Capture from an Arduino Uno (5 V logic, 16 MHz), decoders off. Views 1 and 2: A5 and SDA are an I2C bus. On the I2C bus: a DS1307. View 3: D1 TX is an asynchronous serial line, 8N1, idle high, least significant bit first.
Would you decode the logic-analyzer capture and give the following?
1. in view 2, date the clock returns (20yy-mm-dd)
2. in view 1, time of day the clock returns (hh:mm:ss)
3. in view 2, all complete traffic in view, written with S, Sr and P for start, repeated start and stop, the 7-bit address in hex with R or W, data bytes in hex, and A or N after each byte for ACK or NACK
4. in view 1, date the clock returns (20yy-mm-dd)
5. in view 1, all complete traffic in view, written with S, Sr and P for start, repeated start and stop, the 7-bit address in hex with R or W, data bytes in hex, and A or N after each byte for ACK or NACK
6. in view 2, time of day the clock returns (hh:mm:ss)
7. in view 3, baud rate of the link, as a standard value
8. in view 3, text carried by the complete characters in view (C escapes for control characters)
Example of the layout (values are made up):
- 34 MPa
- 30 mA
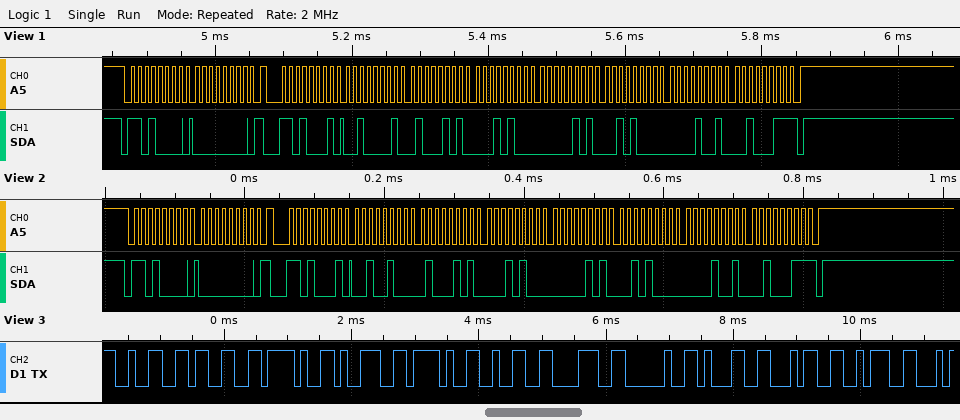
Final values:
- 2023-09-28
- 14:45:21
- S 68W A 00 A Sr 68R A 24 A 45 A 14 A 05 A 28 A 09 A 23 N P
- 2023-09-28
- S 68W A 00 A Sr 68R A 21 A 45 A 14 A 05 A 28 A 09 A 23 N P
- 14:45:24
- 9600 baud
- "23/9/28 14:"
